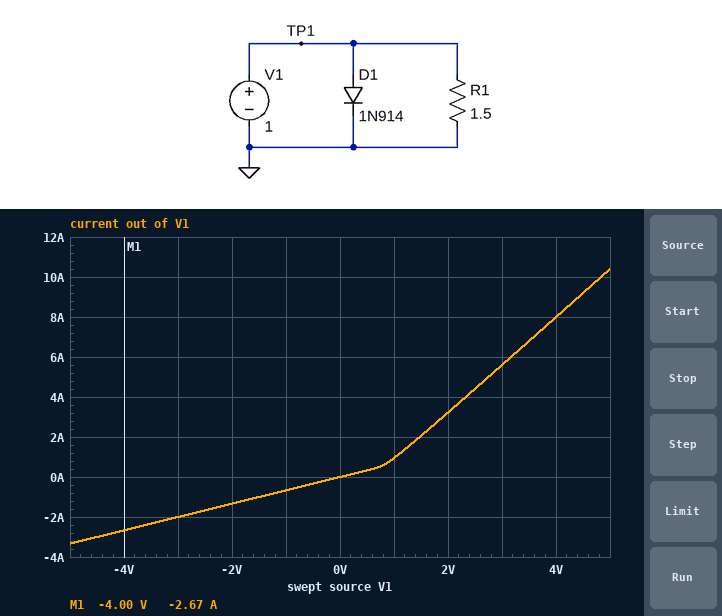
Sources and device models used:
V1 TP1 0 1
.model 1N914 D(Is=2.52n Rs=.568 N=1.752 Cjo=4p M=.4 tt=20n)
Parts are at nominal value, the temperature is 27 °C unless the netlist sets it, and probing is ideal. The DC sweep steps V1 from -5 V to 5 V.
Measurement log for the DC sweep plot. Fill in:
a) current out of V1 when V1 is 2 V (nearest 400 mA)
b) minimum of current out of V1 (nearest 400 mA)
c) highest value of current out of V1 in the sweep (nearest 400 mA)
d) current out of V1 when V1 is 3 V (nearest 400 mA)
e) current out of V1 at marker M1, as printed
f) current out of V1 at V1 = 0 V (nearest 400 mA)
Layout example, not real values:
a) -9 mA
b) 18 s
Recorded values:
a) 3.2 A
b) -3.2 A
c) 10.4 A
d) 5.6 A
e) -2.67 A
f) 0 A
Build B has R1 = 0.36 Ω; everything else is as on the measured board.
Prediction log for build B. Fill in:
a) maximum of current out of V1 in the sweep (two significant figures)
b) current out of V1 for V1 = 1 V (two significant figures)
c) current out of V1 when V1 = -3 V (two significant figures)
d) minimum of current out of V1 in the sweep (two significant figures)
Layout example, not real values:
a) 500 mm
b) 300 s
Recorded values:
a) 21 A
b) 3.1 A
c) -8.3 A
d) -14 A
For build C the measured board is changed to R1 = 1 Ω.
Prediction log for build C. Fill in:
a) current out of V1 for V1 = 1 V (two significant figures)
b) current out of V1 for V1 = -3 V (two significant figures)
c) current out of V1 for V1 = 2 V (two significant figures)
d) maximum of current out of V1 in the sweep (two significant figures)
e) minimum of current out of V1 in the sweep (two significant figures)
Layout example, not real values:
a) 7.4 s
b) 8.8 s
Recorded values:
a) 1.3 A
b) -3.0 A
c) 3.9 A
d) 12 A
e) -5.0 A
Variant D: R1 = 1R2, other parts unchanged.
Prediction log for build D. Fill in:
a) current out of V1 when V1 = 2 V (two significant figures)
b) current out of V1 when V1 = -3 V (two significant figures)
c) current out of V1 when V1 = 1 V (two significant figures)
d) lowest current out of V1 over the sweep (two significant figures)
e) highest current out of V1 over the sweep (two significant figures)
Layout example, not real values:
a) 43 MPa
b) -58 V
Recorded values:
a) 3.6 A
b) -2.5 A
c) 1.1 A
d) -4.2 A
e) 11 A
